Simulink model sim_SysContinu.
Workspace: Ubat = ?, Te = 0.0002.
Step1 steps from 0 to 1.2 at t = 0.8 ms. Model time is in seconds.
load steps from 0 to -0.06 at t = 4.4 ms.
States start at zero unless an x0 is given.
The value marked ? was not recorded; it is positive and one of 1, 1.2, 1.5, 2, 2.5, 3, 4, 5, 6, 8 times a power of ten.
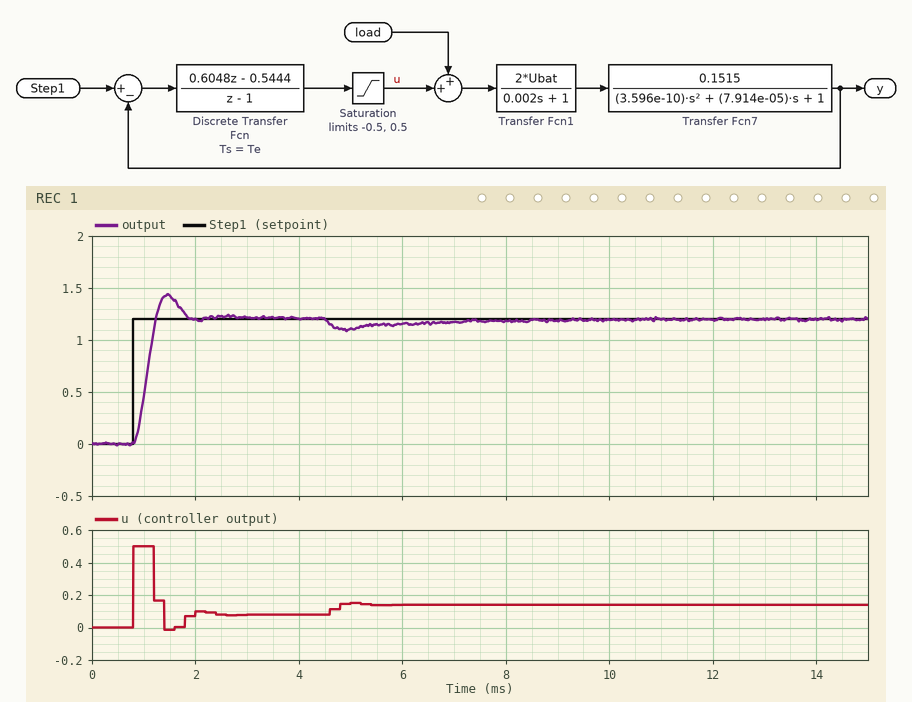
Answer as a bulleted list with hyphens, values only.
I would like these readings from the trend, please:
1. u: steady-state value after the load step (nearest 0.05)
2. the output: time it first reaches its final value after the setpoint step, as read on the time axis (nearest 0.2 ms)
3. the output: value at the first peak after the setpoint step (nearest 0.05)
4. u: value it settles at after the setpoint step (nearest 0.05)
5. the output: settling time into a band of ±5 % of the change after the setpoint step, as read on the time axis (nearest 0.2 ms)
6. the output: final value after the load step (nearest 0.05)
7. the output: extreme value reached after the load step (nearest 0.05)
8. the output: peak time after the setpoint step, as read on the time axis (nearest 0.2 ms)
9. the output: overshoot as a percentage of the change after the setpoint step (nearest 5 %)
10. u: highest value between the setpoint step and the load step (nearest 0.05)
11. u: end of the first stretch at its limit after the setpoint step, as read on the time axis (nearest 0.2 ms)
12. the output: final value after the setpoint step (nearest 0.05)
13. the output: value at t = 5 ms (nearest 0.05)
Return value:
- 0.15
- 1.2 ms
- 1.45
- 0.10
- 1.8 ms
- 1.20
- 1.10
- 1.4 ms
- 20 %
- 0.50
- 1.2 ms
- 1.20
- 1.10
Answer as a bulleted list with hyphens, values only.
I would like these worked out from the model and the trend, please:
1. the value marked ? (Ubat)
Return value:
- 50
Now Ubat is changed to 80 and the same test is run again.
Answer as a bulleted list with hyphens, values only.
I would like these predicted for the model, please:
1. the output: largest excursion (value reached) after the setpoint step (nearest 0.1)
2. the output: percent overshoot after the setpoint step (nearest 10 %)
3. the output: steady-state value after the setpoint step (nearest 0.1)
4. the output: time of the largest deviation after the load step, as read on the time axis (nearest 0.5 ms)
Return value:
- 1.7
- 40 %
- 1.2
- 5.0 ms
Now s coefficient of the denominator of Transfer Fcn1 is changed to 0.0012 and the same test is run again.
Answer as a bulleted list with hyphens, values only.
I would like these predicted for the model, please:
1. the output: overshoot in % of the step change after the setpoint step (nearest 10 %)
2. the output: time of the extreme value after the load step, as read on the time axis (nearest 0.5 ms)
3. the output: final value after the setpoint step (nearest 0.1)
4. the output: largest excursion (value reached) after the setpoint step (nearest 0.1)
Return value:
- 40 %
- 5.0 ms
- 1.2
- 1.6
